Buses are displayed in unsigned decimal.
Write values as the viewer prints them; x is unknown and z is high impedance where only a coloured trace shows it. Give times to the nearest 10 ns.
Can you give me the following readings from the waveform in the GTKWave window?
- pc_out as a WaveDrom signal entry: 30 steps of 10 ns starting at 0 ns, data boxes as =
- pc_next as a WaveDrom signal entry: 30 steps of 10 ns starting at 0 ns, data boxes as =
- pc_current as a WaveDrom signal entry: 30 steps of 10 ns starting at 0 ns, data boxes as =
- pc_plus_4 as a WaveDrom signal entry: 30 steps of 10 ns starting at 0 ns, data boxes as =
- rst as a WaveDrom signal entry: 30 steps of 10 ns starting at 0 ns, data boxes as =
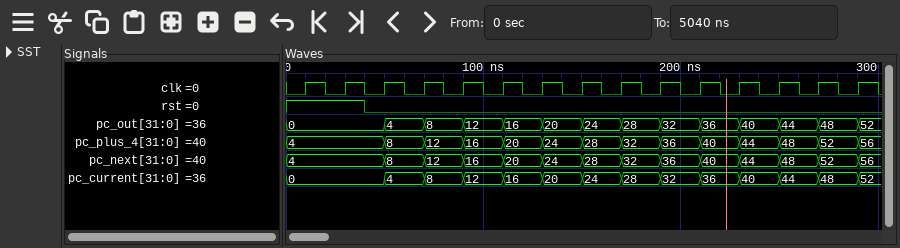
{name: 'pc_out', wave: '=....=.=.=.=.=.=.=.=.=.=.=.=.=', data: '0 4 8 12 16 20 24 28 32 36 40 44 48 52'}
{name: 'pc_next', wave: '=....=.=.=.=.=.=.=.=.=.=.=.=.=', data: '4 8 12 16 20 24 28 32 36 40 44 48 52 56'}
{name: 'pc_current', wave: '=....=.=.=.=.=.=.=.=.=.=.=.=.=', data: '0 4 8 12 16 20 24 28 32 36 40 44 48 52'}
{name: 'pc_plus_4', wave: '=....=.=.=.=.=.=.=.=.=.=.=.=.=', data: '4 8 12 16 20 24 28 32 36 40 44 48 52 56'}
{name: 'rst', wave: '1...0.........................'}
